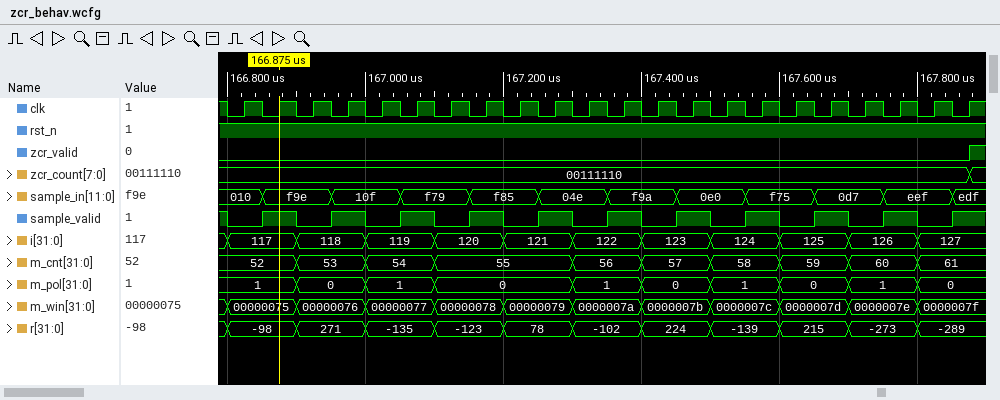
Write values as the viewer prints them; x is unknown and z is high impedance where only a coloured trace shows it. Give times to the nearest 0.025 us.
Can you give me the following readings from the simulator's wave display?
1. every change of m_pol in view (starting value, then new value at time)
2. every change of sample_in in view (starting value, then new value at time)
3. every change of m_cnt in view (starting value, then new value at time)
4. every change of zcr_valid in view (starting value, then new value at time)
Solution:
1, 0 at 166.9 us, 1 at 167 us, 0 at 167.1 us, 1 at 167.3 us, 0 at 167.4 us, 1 at 167.5 us, 0 at 167.6 us, 1 at 167.7 us, 0 at 167.8 us
010, f9e at 166.85 us, 10f at 166.95 us, f79 at 167.05 us, f85 at 167.15 us, 04e at 167.25 us, f9a at 167.35 us, 0e0 at 167.45 us, f75 at 167.55 us, 0d7 at 167.65 us, eef at 167.75 us, edf at 167.85 us
52, 53 at 166.9 us, 54 at 167 us, 55 at 167.1 us, 56 at 167.3 us, 57 at 167.4 us, 58 at 167.5 us, 59 at 167.6 us, 60 at 167.7 us, 61 at 167.8 us
0, 1 at 167.875 us
